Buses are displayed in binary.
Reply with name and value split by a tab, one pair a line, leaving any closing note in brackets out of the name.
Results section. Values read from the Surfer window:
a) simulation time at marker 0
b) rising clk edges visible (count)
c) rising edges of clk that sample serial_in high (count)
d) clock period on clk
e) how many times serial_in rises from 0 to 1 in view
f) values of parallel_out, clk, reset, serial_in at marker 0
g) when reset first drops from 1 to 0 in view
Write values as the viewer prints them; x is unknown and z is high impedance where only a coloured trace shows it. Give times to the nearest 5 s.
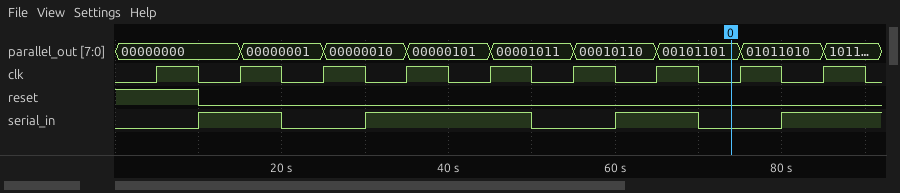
simulation time at marker 0	75 s
rising clk edges visible	9
rising edges of clk that sample serial_in high	5
clock period on clk	10 s
how many times serial_in rises from 0 to 1 in view	4
values of parallel_out, clk, reset, serial_in at marker 0	parallel_out=00101101, clk=0, reset=0, serial_in=0
when reset first drops from 1 to 0 in view	10 s
